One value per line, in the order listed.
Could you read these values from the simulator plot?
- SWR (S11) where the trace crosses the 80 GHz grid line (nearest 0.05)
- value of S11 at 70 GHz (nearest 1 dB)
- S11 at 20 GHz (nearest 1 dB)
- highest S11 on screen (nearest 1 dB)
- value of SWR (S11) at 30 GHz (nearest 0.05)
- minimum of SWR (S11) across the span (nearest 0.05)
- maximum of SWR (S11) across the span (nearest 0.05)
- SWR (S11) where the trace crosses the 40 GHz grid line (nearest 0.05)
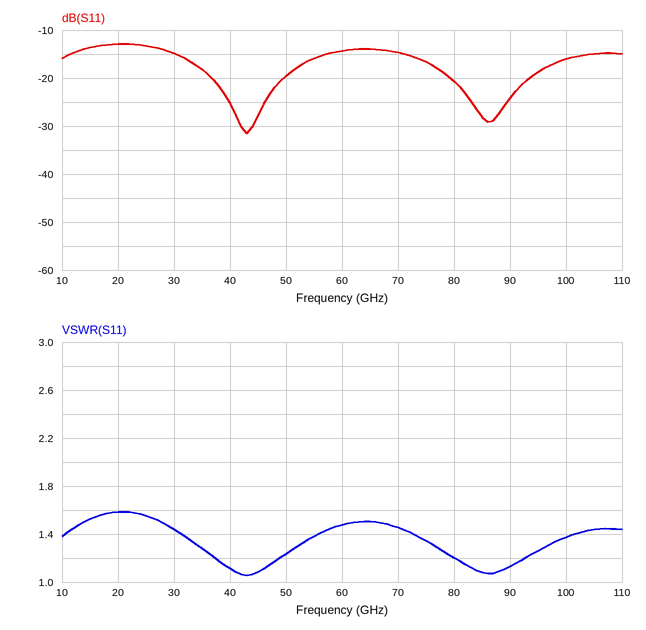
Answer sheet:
1.20
-15 dB
-13 dB
-13 dB
1.45
1.05
1.60
1.10
